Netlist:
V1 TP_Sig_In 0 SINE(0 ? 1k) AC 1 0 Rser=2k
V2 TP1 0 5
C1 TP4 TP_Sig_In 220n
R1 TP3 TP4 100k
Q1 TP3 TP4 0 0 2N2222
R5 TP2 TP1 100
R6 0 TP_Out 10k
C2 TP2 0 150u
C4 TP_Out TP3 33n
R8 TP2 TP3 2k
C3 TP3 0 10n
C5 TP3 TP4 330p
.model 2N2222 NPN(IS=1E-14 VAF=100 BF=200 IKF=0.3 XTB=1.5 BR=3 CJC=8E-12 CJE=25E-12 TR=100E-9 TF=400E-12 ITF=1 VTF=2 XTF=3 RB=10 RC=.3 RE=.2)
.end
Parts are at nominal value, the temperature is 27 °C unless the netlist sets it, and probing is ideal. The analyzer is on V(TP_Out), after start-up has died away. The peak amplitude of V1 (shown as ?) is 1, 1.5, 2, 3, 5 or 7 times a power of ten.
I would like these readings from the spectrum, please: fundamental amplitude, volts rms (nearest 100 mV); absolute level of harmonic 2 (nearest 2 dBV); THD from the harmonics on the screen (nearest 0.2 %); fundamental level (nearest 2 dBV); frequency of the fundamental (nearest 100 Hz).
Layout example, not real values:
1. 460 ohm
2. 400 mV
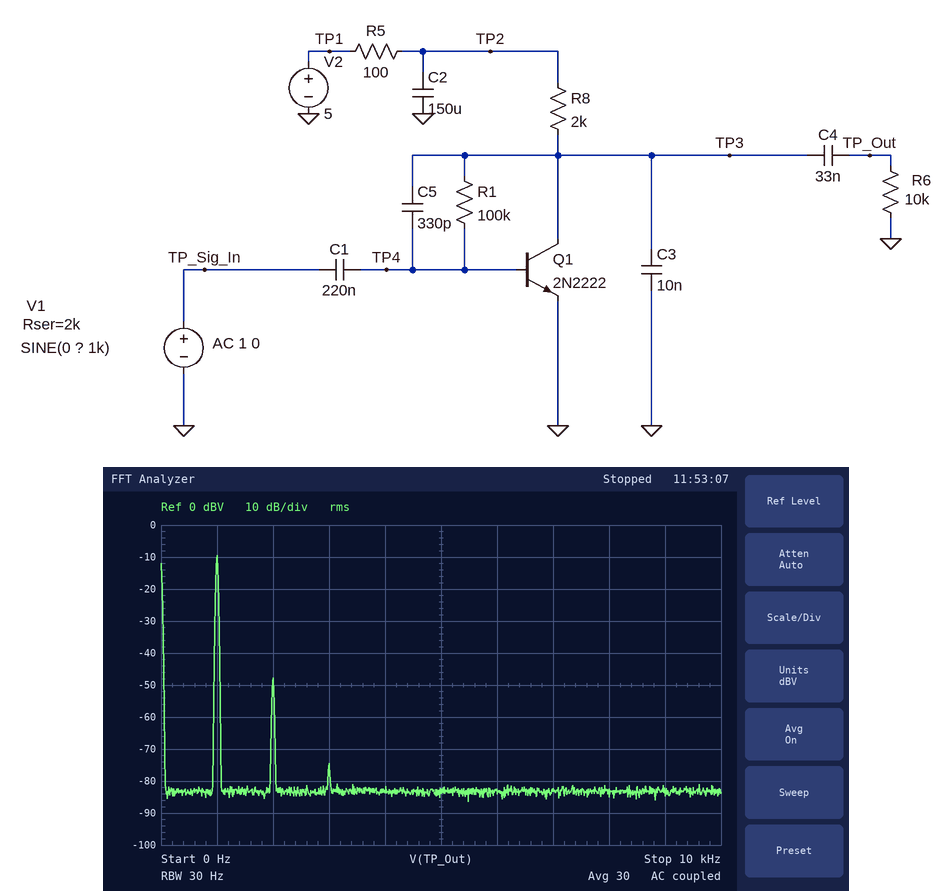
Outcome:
1. 300 mV
2. -48 dBV
3. 1.2 %
4. -10 dBV
5. 1.0 kHz
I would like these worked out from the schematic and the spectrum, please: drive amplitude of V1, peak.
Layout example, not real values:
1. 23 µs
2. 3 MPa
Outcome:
1. 20 mV
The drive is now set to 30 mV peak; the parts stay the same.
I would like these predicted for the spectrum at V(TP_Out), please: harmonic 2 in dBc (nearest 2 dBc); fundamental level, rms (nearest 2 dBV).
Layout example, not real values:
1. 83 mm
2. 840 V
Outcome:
1. -34 dBc
2. -6 dBV
